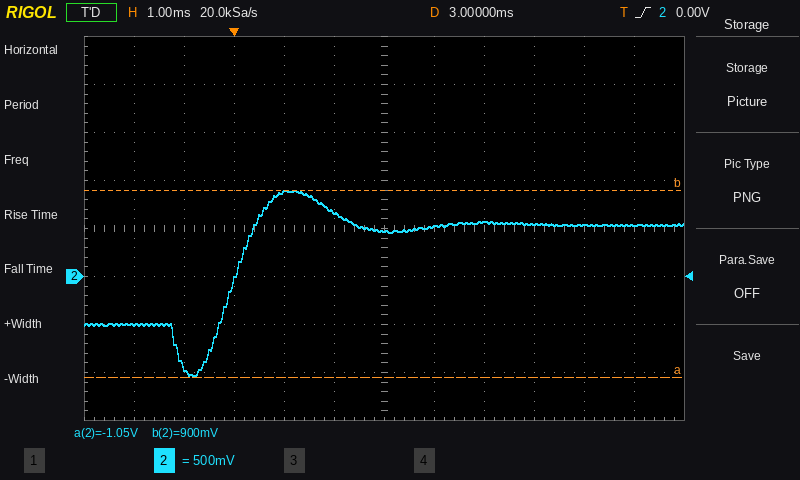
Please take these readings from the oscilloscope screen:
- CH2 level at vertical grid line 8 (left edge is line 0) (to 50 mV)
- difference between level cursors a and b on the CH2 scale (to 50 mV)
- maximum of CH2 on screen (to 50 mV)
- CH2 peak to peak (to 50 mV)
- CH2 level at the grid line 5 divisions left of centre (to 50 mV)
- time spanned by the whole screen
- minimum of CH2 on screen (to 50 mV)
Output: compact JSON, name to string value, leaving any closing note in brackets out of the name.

{"CH2 level at vertical grid line 8 (left edge is line 0)": "550 mV", "difference between level cursors a and b on the CH2 scale": "1.95 V", "maximum of CH2 on screen": "900 mV", "CH2 peak to peak": "1.95 V", "CH2 level at the grid line 5 divisions left of centre": "-500 mV", "time spanned by the whole screen": "12 ms", "minimum of CH2 on screen": "-1.05 V"}
